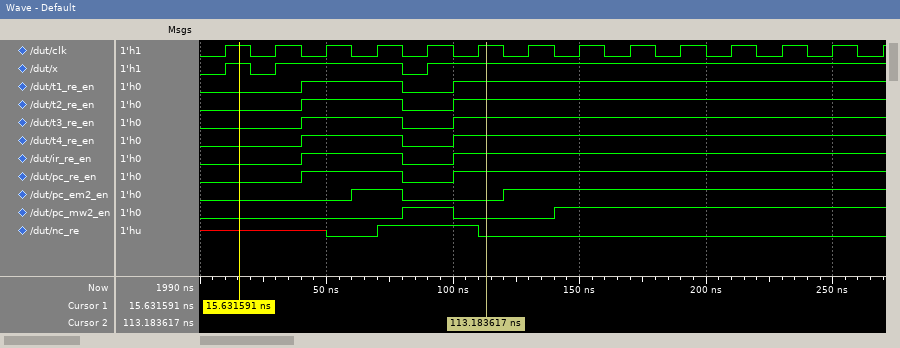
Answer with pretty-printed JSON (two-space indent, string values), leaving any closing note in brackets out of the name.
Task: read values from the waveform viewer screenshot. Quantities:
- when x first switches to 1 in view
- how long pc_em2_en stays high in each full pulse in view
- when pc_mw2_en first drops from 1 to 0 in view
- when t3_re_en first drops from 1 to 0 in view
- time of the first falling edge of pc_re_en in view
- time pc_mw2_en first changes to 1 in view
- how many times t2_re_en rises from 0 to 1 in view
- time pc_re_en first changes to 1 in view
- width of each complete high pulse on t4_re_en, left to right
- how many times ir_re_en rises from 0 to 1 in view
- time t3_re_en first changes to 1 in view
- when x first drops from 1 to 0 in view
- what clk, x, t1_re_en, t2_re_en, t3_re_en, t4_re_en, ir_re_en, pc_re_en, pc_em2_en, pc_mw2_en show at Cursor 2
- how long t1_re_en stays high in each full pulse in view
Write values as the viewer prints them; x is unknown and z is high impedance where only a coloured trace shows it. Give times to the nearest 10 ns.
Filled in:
{
  "when x first switches to 1 in view": "10 ns",
  "how long pc_em2_en stays high in each full pulse in view": "20 ns",
  "when pc_mw2_en first drops from 1 to 0 in view": "100 ns",
  "when t3_re_en first drops from 1 to 0 in view": "80 ns",
  "time of the first falling edge of pc_re_en in view": "80 ns",
  "time pc_mw2_en first changes to 1 in view": "80 ns",
  "how many times t2_re_en rises from 0 to 1 in view": "2",
  "time pc_re_en first changes to 1 in view": "40 ns",
  "width of each complete high pulse on t4_re_en, left to right": "40 ns",
  "how many times ir_re_en rises from 0 to 1 in view": "2",
  "time t3_re_en first changes to 1 in view": "40 ns",
  "when x first drops from 1 to 0 in view": "20 ns",
  "what clk, x, t1_re_en, t2_re_en, t3_re_en, t4_re_en, ir_re_en, pc_re_en, pc_em2_en, pc_mw2_en show at Cursor 2": "clk=1, x=1, t1_re_en=1, t2_re_en=1, t3_re_en=1, t4_re_en=1, ir_re_en=1, pc_re_en=1, pc_em2_en=0, pc_mw2_en=0",
  "how long t1_re_en stays high in each full pulse in view": "40 ns"
}
